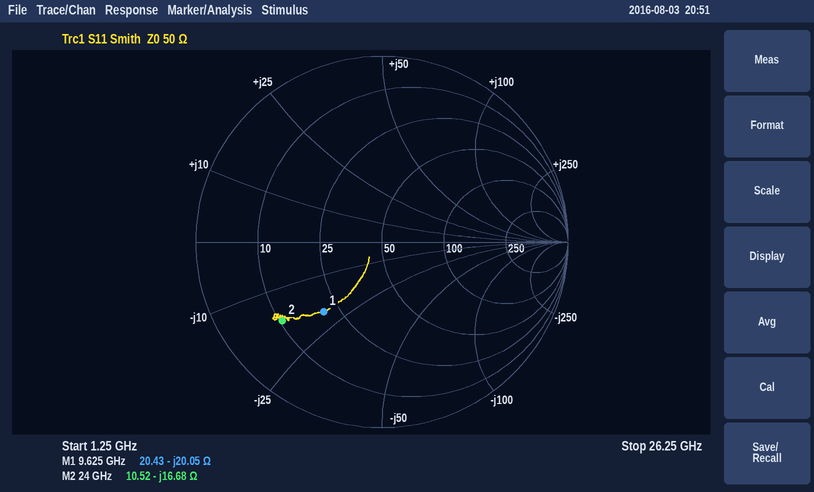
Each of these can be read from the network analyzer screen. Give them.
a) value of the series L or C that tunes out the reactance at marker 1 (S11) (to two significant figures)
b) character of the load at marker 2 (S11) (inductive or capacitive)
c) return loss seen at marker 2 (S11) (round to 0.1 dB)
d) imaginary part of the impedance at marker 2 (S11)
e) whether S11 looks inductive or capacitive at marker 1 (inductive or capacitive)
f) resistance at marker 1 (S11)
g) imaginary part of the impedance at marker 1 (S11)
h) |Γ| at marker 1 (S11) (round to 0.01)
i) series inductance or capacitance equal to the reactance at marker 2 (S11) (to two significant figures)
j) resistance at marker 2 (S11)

330 pH
capacitive
3.3 dB
-16.68 Ω
capacitive
20.43 Ω
-20.05 Ω
0.49
400 fF
10.52 Ω
